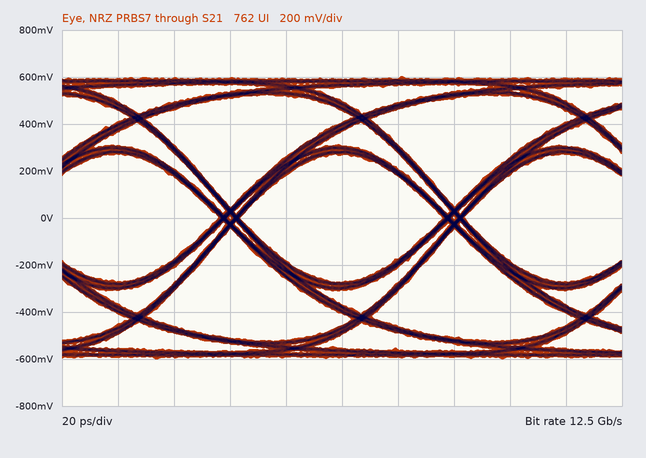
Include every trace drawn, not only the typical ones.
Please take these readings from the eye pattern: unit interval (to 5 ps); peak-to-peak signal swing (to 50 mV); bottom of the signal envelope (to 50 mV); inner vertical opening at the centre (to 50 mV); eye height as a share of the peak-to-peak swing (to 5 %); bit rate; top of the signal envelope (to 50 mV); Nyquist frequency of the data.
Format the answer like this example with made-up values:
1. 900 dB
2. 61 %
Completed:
1. 80 ps
2. 1.20 V
3. -600 mV
4. 550 mV
5. 45 %
6. 12.5 Gb/s
7. 600 mV
8. 6.25 GHz
